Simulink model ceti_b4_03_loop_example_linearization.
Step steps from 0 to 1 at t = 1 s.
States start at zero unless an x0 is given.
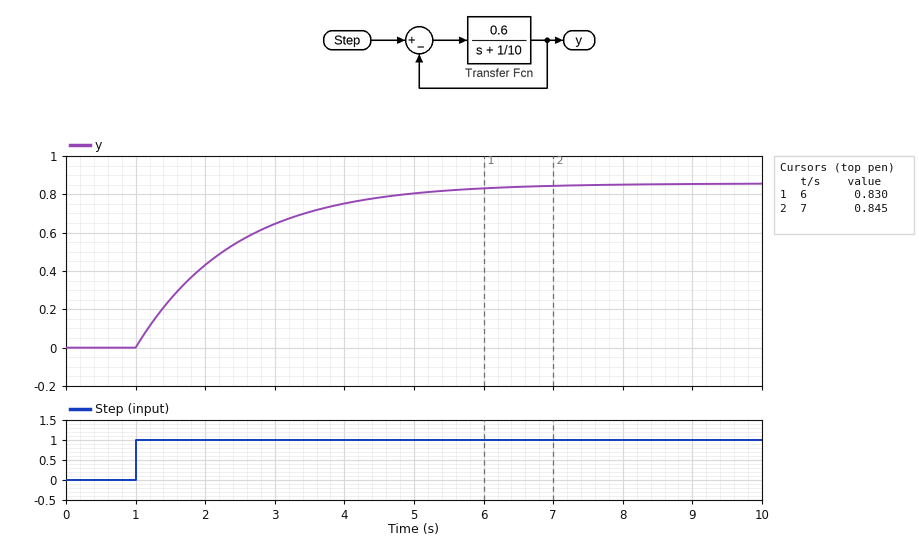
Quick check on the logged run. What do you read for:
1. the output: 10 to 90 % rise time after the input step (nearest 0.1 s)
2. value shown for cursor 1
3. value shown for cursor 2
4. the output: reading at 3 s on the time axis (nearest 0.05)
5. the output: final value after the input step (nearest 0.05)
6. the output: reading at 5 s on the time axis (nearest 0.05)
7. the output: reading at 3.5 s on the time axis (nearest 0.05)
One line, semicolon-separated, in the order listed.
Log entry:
3.1 s; 0.830; 0.845; 0.65; 0.85; 0.80; 0.70
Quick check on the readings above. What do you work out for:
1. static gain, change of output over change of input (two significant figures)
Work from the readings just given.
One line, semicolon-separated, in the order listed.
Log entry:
0.85
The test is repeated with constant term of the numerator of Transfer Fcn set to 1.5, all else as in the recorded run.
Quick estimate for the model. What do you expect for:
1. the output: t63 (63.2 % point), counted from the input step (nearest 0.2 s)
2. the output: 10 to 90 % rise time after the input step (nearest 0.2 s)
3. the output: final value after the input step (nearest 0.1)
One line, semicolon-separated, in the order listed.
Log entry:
0.6 s; 1.4 s; 0.9
